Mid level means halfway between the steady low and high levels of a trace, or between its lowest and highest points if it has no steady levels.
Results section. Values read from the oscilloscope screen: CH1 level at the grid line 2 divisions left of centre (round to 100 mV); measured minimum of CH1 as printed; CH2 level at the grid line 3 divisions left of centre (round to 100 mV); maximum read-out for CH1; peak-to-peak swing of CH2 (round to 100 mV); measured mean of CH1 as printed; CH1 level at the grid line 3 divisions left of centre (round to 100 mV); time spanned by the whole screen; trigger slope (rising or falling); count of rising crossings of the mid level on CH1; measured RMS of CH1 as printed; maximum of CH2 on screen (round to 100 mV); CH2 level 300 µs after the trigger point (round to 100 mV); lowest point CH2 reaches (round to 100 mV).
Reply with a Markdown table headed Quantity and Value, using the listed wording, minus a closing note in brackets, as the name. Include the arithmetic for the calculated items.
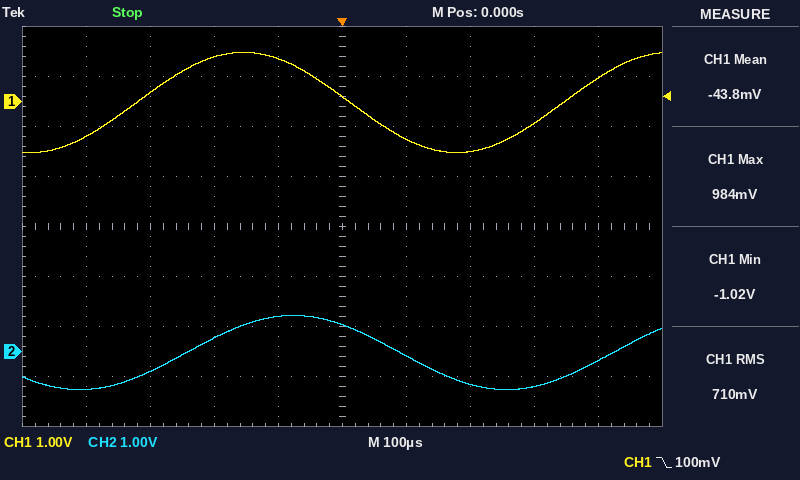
| Quantity | Value |
|---|---|
| CH1 level at the grid line 2 divisions left of centre | 900 mV |
| measured minimum of CH1 as printed | -1.02 V |
| CH2 level at the grid line 3 divisions left of centre | -400 mV |
| maximum read-out for CH1 | 984 mV |
| peak-to-peak swing of CH2 | 700 mV − (-800 mV) = 1.5 V |
| measured mean of CH1 as printed | -43.8 mV |
| CH1 level at the grid line 3 divisions left of centre | 200 mV |
| time spanned by the whole screen | 1 ms |
| trigger slope | falling |
| count of rising crossings of the mid level on CH1 | 2 |
| measured RMS of CH1 as printed | 710 mV |
| maximum of CH2 on screen | 700 mV |
| CH2 level 300 µs after the trigger point | -700 mV |
| lowest point CH2 reaches | -800 mV |
